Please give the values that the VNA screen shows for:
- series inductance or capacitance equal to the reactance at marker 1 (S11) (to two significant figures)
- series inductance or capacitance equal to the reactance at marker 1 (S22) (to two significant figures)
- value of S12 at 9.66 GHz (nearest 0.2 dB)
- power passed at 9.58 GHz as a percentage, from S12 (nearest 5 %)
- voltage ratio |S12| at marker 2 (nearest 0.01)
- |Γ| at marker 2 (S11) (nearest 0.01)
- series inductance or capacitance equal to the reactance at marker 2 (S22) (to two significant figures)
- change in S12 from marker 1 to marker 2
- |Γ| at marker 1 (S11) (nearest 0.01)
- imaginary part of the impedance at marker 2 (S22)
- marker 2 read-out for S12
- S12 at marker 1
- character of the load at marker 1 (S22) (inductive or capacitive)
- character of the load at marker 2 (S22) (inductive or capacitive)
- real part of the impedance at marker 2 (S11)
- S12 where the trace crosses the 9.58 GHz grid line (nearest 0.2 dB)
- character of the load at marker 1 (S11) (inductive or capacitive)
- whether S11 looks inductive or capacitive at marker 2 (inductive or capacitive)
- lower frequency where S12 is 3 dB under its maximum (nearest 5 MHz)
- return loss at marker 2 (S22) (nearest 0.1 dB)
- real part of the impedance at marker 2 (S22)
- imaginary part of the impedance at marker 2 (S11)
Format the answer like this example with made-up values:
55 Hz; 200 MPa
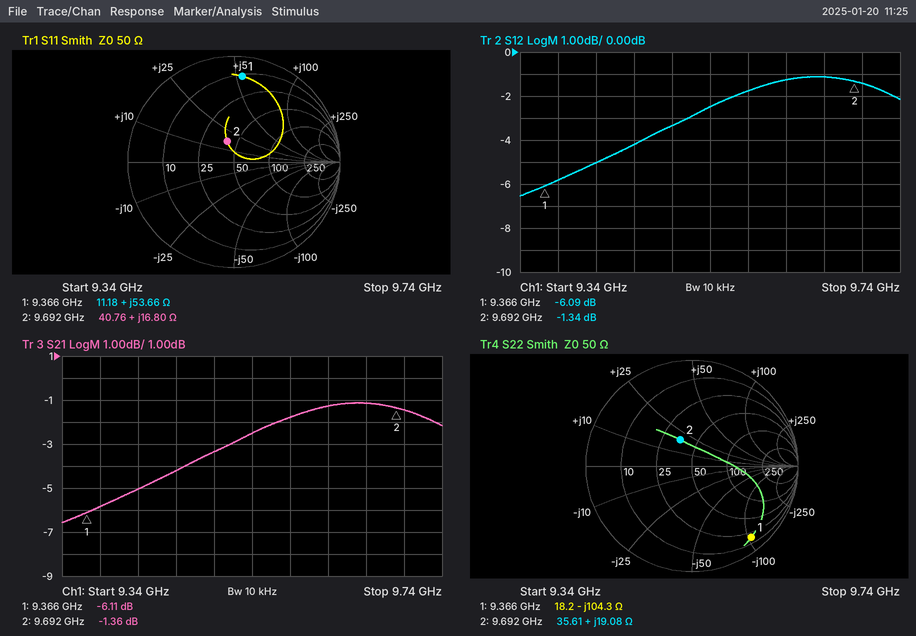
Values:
910 pH; 160 fF; -1.2 dB; 65 %; 0.86; 0.21; 310 pH; 4.75 dB; 0.81; +19.08 Ω; -1.34 dB; -6.09 dB; capacitive; inductive; 40.76 Ω; -1.8 dB; inductive; inductive; 9.465 GHz; 11.3 dB; 35.61 Ω; +16.80 Ω
